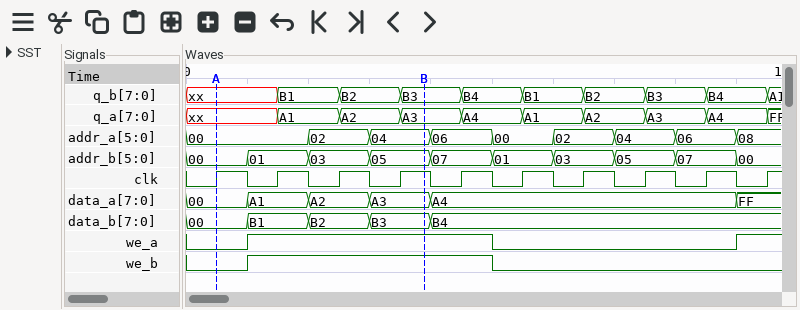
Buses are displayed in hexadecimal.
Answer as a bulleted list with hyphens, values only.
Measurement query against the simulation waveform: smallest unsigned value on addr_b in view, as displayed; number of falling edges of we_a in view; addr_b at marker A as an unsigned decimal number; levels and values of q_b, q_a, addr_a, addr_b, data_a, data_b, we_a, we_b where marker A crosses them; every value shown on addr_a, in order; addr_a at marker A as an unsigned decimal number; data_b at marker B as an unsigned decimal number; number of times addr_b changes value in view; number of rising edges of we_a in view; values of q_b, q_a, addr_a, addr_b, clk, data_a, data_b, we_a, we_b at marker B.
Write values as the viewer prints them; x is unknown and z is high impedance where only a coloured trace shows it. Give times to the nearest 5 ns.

- 00
- 1
- 0
- q_b=xx, q_a=xx, addr_a=00, addr_b=00, data_a=00, data_b=00, we_a=0, we_b=0
- 00, 02, 04, 06, 00, 02, 04, 06, 08
- 0
- 179
- 9
- 2
- q_b=B3, q_a=A3, addr_a=04, addr_b=05, clk=1, data_a=A3, data_b=B3, we_a=1, we_b=1
